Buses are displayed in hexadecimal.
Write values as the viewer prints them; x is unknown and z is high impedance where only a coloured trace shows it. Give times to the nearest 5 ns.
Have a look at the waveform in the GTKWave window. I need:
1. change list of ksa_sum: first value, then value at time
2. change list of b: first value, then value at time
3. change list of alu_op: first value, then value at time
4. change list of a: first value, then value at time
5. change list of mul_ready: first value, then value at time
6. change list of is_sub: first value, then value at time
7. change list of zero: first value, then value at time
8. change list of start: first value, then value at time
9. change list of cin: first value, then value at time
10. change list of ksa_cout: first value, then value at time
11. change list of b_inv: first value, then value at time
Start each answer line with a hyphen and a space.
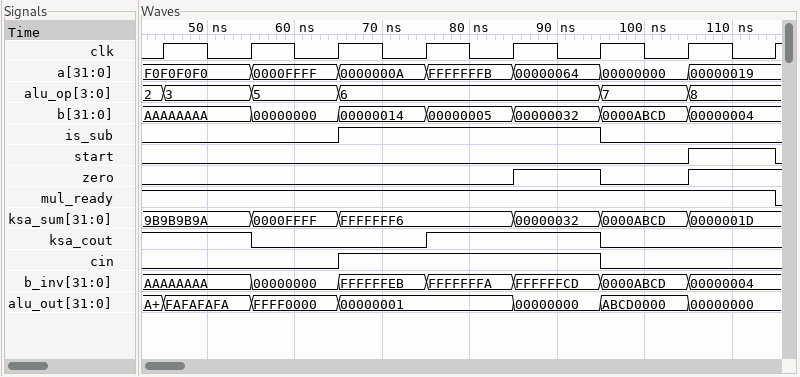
- 9B9B9B9A, 0000FFFF at 55 ns, FFFFFFF6 at 65 ns, 00000032 at 85 ns, 0000ABCD at 95 ns, 0000001D at 105 ns
- AAAAAAAA, 00000000 at 55 ns, 00000014 at 65 ns, 00000005 at 75 ns, 00000032 at 85 ns, 0000ABCD at 95 ns, 00000004 at 105 ns
- 2, 3 at 45 ns, 5 at 55 ns, 6 at 65 ns, 7 at 95 ns, 8 at 105 ns
- F0F0F0F0, 0000FFFF at 55 ns, 0000000A at 65 ns, FFFFFFFB at 75 ns, 00000064 at 85 ns, 00000000 at 95 ns, 00000019 at 105 ns
- 1, 0 at 115 ns
- 0, 1 at 65 ns, 0 at 95 ns
- 0, 1 at 85 ns, 0 at 95 ns, 1 at 105 ns
- 0, 1 at 105 ns, 0 at 115 ns
- 0, 1 at 65 ns, 0 at 95 ns
- 1, 0 at 55 ns, 1 at 75 ns, 0 at 95 ns
- AAAAAAAA, 00000000 at 55 ns, FFFFFFEB at 65 ns, FFFFFFFA at 75 ns, FFFFFFCD at 85 ns, 0000ABCD at 95 ns, 00000004 at 105 ns
